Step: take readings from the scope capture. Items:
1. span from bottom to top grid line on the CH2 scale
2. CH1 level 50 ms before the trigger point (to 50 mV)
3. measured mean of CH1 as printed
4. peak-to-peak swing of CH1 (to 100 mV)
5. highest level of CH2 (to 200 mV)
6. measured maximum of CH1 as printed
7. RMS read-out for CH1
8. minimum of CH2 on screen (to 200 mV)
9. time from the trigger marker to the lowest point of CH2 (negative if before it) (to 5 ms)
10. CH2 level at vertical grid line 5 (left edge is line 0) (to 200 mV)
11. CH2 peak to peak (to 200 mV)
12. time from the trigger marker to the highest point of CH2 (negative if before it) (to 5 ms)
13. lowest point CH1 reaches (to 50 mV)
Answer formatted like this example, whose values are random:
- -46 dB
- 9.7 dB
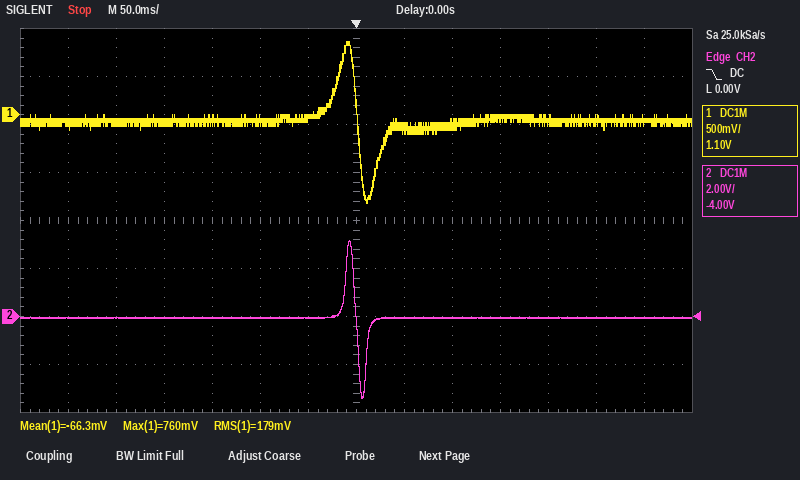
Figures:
- 16 V
- -50 mV
- -66.3 mV
- 1.70 V
- 3.2 V
- 760 mV
- 179 mV
- -3.4 V
- +5 ms
- 0.0 V
- 6.6 V
- -5 ms
- -900 mV
